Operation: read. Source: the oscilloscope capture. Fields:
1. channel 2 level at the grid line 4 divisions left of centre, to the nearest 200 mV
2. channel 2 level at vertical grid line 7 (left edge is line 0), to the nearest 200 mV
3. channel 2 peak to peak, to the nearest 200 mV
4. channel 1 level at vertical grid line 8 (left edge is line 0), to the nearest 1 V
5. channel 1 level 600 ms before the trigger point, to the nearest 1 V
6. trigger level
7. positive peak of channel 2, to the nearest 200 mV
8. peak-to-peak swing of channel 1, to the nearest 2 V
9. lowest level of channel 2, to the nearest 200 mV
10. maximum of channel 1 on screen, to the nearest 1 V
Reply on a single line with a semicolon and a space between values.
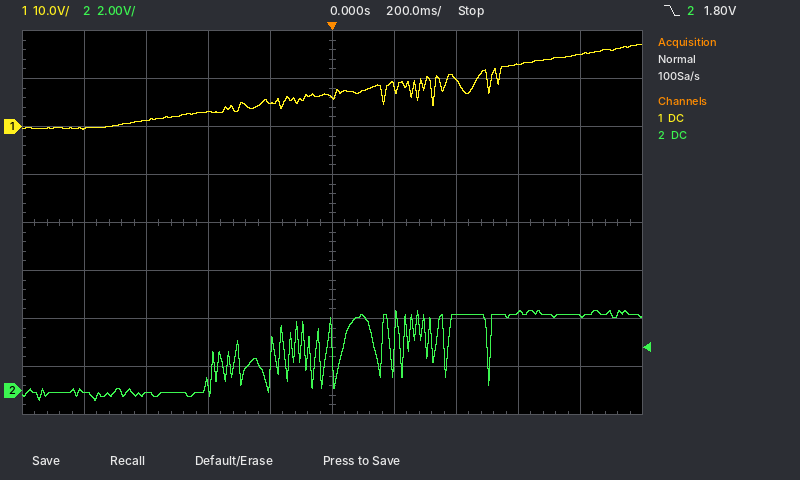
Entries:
0.0 V; 3.2 V; 3.8 V; 13 V; 1 V; 1.80 V; 3.4 V; 18 V; -400 mV; 17 V
